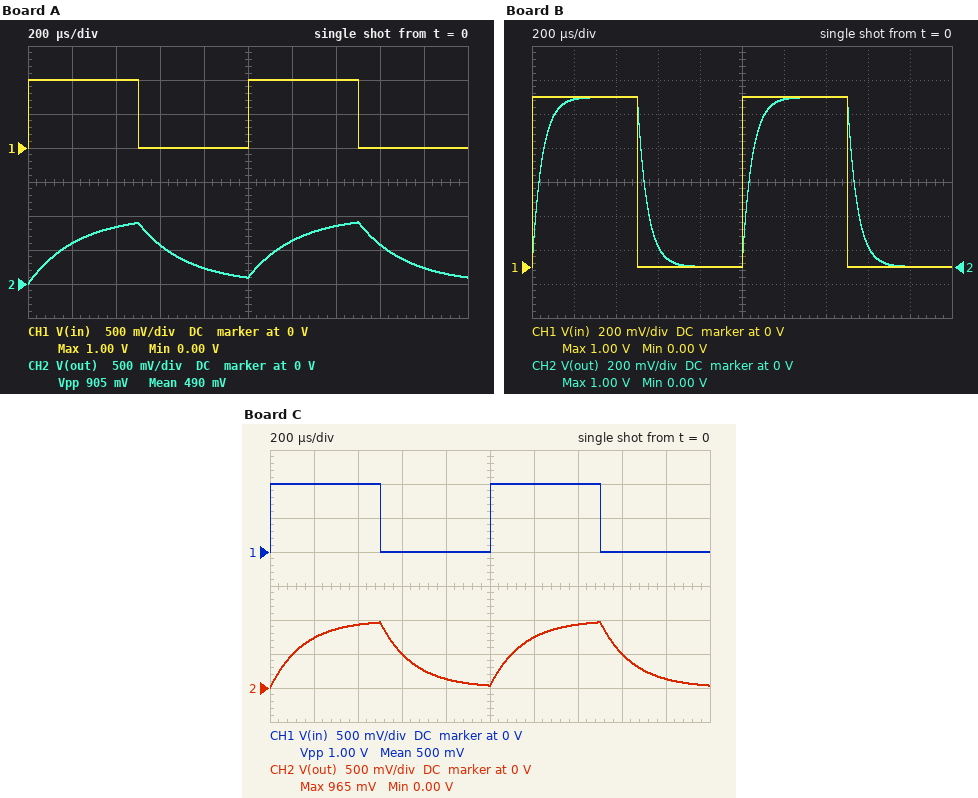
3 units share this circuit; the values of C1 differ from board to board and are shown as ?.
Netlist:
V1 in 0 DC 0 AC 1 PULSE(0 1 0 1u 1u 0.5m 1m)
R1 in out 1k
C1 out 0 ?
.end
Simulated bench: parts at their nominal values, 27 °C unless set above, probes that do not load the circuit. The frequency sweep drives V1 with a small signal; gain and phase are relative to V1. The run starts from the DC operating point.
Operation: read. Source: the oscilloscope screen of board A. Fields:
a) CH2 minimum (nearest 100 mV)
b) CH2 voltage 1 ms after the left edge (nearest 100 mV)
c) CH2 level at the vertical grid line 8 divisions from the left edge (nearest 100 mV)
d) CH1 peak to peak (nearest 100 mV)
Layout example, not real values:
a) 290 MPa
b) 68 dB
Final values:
a) 0 V
b) 100 mV
c) 600 mV
d) 1.0 V
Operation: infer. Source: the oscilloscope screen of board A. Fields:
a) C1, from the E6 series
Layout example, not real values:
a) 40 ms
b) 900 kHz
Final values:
a) 220 nF
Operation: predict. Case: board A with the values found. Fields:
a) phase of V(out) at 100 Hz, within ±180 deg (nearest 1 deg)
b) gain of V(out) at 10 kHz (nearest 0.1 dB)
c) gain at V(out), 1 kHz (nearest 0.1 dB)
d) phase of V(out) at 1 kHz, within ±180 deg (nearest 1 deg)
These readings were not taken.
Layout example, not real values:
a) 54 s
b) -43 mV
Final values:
a) -8 deg
b) -22.8 dB
c) -4.6 dB
d) -54 deg
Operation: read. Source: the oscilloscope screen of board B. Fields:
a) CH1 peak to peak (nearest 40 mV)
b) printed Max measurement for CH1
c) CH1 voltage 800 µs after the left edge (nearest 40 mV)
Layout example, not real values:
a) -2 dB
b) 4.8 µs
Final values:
a) 1.00 V
b) 1.00 V
c) 0 V
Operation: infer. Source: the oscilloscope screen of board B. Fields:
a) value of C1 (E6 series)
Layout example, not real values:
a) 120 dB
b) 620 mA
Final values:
a) 47 nF
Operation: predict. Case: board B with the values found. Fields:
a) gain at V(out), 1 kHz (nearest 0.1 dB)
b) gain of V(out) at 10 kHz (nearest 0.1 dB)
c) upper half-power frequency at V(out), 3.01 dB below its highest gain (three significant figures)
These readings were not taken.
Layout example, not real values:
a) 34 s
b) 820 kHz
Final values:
a) -0.4 dB
b) -9.9 dB
c) 3.39 kHz
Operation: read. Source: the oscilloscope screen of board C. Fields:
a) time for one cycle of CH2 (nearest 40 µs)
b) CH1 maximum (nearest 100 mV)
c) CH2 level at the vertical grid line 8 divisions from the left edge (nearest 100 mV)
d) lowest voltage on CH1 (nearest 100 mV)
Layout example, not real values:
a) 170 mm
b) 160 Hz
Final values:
a) 1.00 ms
b) 1.0 V
c) 500 mV
d) 0 V
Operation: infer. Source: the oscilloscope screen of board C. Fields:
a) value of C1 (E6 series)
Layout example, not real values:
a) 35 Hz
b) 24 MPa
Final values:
a) 150 nF
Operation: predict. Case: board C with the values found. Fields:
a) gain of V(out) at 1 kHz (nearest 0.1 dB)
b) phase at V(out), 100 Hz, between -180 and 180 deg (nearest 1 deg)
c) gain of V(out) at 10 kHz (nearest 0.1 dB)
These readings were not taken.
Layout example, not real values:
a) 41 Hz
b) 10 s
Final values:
a) -2.8 dB
b) -5 deg
c) -19.5 dB
